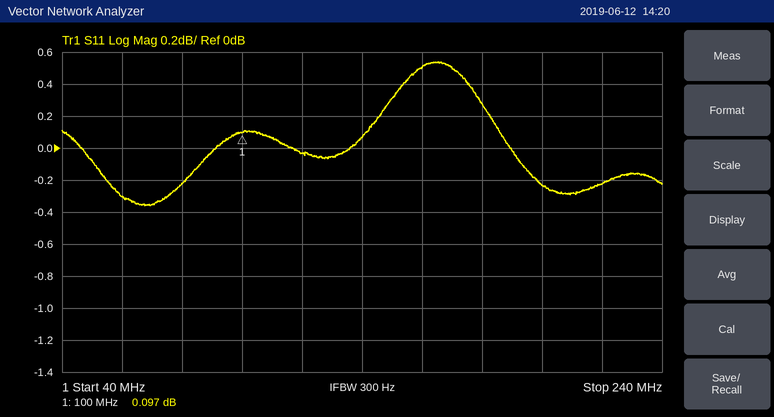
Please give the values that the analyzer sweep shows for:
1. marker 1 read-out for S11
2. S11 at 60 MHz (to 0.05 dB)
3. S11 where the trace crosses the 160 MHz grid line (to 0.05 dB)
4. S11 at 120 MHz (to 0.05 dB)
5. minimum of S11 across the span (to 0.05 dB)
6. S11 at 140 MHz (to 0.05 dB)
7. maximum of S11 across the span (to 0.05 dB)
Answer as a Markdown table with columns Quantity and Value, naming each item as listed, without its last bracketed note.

| Quantity | Value |
|---|---|
| marker 1 read-out for S11 | 0.097 dB |
| S11 at 60 MHz | -0.30 dB |
| S11 where the trace crosses the 160 MHz grid line | 0.50 dB |
| S11 at 120 MHz | -0.05 dB |
| minimum of S11 across the span | -0.35 dB |
| S11 at 140 MHz | 0.05 dB |
| maximum of S11 across the span | 0.55 dB |
